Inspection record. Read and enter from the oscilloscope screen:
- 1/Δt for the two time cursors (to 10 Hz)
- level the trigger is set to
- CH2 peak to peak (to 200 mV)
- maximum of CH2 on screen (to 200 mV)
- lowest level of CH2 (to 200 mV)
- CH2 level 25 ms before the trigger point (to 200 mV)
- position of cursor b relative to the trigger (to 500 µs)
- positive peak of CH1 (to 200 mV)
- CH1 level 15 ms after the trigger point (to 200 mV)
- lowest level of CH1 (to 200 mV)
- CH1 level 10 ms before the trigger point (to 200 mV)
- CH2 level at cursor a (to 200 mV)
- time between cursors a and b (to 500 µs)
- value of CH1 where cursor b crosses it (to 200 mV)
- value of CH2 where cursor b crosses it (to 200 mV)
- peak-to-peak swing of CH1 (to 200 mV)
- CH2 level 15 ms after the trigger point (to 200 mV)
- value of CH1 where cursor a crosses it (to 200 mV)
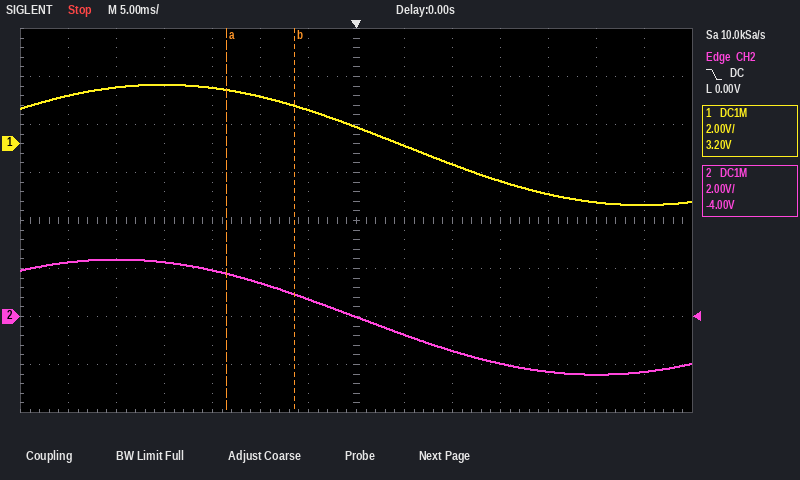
140 Hz
0.00 V
4.8 V
2.4 V
-2.4 V
2.4 V
-6.5 ms
2.4 V
-1.6 V
-2.6 V
2.0 V
1.8 V
7.0 ms
1.6 V
1.0 V
5.0 V
-2.0 V
2.2 V
